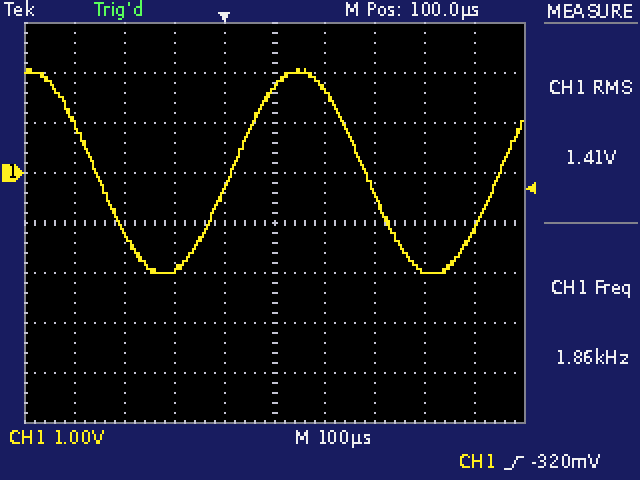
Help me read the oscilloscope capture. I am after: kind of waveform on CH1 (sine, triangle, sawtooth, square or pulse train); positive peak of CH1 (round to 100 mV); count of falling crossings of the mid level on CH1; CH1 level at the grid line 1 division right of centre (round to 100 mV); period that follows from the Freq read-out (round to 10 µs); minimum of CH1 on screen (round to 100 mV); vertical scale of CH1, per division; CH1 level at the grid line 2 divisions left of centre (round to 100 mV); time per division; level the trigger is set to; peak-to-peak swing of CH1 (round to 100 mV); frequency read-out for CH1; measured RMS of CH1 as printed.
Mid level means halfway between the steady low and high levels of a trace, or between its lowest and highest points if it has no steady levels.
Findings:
sine
2.1 V
2
1.7 V
540 µs
-2.0 V
1 V
-1.9 V
100 µs
-320 mV
4.1 V
1.86 kHz
1.41 V
